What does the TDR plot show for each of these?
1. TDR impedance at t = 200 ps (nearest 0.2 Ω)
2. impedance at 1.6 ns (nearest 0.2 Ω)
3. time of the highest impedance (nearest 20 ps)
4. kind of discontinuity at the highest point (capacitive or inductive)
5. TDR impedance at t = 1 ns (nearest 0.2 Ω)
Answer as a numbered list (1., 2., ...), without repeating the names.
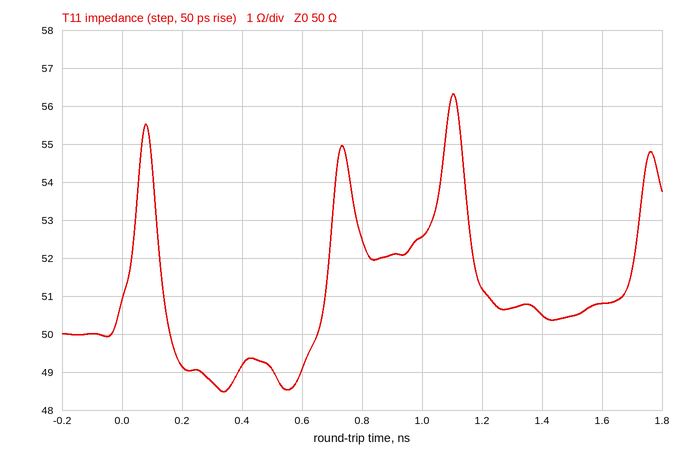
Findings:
1. 49.2 Ω
2. 50.8 Ω
3. 1.10 ns
4. inductive
5. 52.6 Ω
